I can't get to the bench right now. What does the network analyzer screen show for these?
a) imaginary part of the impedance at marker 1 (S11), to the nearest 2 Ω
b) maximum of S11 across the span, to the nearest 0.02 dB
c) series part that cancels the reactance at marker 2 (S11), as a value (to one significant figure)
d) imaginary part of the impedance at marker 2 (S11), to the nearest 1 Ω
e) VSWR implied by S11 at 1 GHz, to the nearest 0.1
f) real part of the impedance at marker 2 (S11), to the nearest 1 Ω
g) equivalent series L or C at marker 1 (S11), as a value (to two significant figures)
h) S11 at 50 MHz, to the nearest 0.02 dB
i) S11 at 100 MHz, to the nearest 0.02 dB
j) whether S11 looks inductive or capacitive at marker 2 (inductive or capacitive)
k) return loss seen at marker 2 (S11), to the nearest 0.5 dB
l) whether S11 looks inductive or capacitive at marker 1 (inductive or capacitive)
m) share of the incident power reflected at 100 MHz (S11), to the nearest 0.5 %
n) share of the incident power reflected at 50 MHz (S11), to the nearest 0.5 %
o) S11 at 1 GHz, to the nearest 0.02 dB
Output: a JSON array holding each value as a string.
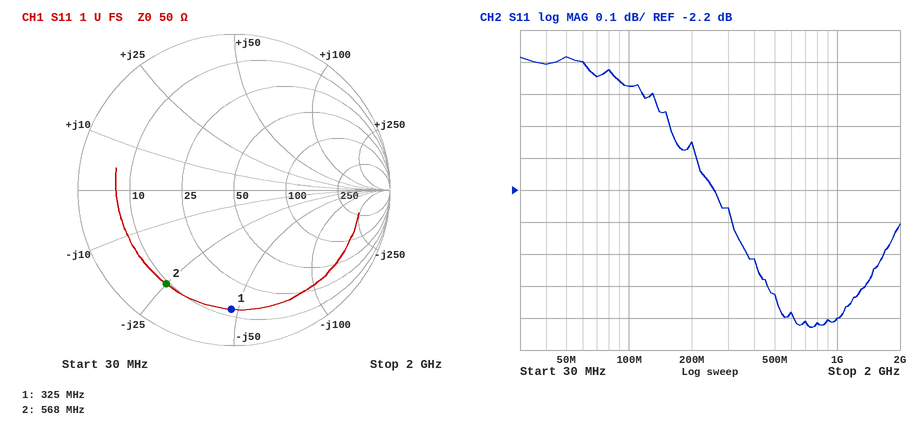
["-48 Ω", "-1.78 dB", "7 nH", "-25 Ω", "6.7", "9 Ω", "10 pF", "-1.78 dB", "-1.88 dB", "capacitive", "2.5 dB", "capacitive", "65.0 %", "66.5 %", "-2.60 dB"]
